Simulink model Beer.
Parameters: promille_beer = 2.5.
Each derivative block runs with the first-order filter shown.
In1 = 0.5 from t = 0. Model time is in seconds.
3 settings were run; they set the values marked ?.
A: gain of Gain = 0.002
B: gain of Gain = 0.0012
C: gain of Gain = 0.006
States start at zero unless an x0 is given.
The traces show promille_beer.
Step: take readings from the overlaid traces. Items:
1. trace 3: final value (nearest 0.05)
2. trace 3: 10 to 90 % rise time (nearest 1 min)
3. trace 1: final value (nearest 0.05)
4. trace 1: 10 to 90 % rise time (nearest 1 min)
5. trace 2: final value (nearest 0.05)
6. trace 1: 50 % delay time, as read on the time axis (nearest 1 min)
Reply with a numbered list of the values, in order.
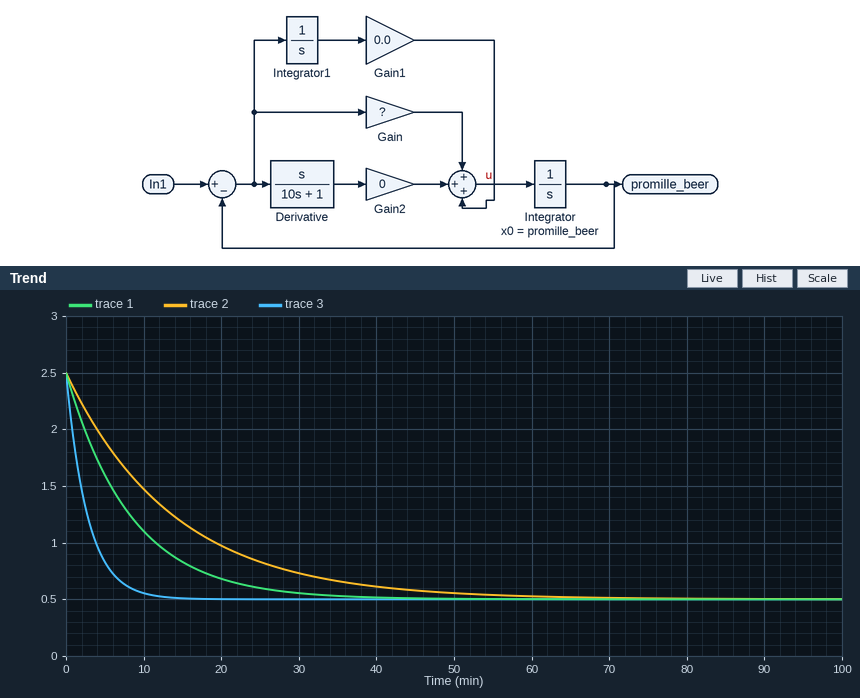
1. 0.50
2. 6 min
3. 0.50
4. 18 min
5. 0.50
6. 6 min
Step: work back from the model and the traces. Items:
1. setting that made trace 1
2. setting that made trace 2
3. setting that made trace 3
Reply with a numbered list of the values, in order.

1. A
2. B
3. C
